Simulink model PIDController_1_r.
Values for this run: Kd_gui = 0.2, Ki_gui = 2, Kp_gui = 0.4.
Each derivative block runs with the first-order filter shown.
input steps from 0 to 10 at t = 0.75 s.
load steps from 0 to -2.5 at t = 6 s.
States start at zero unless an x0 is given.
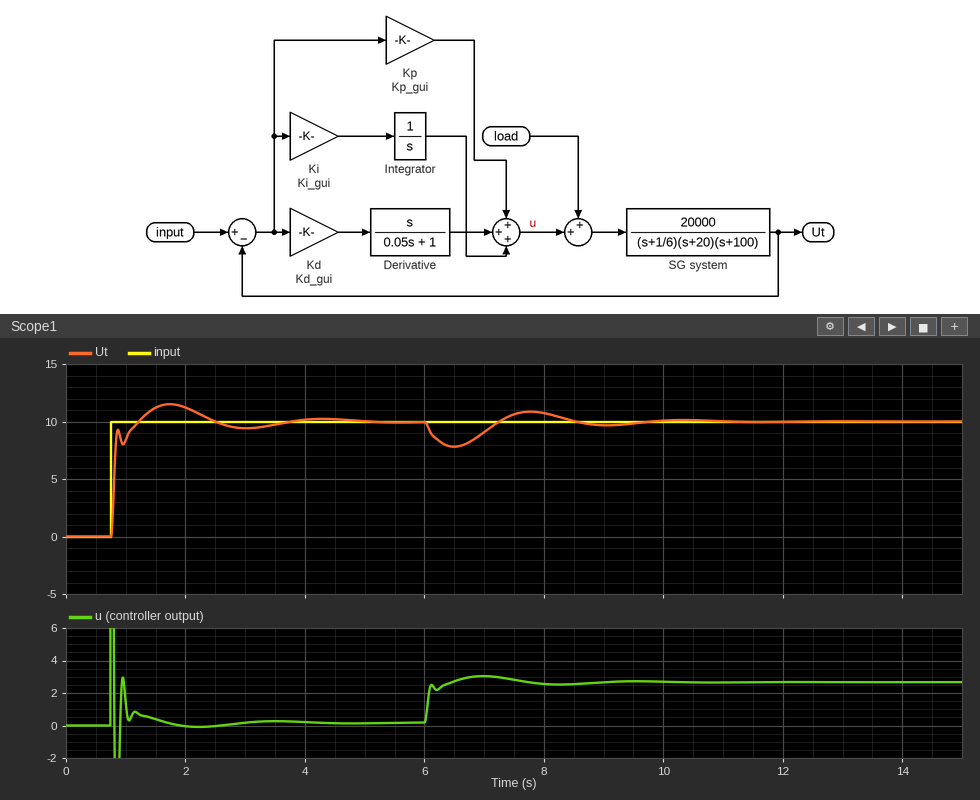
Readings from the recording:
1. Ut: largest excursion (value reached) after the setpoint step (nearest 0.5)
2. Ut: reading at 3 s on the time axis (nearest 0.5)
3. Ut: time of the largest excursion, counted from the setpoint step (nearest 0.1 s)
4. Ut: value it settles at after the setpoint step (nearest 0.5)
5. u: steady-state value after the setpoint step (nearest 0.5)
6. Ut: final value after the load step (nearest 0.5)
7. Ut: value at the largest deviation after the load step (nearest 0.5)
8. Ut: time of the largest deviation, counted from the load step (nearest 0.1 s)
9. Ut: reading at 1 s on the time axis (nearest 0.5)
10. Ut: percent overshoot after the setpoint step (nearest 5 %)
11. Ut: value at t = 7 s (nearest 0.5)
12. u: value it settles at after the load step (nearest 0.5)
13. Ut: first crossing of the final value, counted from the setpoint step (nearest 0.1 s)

11.5
9.5
1.0 s
10.0
0.0
10.0
8.0
0.5 s
8.5
15 %
9.0
2.5
0.5 s
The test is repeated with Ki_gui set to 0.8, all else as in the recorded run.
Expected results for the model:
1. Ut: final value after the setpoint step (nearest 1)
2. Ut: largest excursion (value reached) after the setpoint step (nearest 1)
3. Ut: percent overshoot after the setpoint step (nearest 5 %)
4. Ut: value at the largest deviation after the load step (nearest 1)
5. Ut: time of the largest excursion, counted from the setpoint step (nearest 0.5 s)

10
11
10 %
7
1.5 s
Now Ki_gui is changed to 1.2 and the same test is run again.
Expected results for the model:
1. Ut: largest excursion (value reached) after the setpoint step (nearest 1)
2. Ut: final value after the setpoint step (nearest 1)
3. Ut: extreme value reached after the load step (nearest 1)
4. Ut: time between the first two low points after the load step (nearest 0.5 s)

11
10
7
3.5 s
